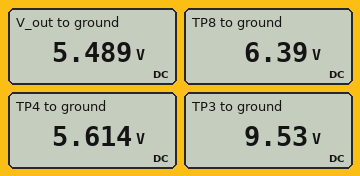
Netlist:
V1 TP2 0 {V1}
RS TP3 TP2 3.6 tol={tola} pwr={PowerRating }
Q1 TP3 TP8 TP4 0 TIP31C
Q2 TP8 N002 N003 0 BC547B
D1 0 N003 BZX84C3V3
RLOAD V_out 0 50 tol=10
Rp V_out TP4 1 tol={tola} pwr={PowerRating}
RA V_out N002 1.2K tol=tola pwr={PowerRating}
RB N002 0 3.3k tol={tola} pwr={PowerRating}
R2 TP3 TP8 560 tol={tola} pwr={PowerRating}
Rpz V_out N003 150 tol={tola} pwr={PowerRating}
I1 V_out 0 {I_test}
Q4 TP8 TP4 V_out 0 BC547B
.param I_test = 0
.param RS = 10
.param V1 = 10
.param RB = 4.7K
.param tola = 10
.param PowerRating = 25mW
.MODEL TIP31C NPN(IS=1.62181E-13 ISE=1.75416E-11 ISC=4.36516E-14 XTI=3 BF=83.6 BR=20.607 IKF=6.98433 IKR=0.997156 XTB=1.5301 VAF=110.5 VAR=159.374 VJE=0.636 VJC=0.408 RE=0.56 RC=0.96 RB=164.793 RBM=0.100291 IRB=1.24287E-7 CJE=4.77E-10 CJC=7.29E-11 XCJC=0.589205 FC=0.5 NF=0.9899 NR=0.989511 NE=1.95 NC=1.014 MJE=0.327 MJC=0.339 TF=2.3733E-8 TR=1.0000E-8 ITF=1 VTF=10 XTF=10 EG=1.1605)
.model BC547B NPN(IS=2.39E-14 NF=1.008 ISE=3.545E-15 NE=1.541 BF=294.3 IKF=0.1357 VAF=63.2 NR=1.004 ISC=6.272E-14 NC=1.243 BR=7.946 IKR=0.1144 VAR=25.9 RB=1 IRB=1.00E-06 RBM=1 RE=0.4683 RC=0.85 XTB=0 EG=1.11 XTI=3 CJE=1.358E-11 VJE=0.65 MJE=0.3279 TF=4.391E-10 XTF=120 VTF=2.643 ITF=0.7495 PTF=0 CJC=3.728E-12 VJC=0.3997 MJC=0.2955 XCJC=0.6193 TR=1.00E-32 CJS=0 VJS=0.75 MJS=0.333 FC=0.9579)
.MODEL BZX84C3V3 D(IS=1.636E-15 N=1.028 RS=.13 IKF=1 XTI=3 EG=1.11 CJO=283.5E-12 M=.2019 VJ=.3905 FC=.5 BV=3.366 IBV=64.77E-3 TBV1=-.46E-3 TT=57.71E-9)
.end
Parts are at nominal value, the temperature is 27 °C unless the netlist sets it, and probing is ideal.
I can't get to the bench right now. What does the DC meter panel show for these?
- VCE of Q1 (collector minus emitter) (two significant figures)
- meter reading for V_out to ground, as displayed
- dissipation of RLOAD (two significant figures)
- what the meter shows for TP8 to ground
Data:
3.9 V
5.489 V
600 mW
6.39 V
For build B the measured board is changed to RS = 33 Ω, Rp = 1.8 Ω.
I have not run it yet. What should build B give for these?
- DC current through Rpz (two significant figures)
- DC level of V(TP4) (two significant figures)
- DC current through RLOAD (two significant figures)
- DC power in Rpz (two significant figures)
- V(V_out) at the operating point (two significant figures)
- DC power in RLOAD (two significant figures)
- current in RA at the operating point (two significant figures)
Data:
9.9 mA
5.0 V
96 mA
15 mW
4.8 V
460 mW
1.1 mA
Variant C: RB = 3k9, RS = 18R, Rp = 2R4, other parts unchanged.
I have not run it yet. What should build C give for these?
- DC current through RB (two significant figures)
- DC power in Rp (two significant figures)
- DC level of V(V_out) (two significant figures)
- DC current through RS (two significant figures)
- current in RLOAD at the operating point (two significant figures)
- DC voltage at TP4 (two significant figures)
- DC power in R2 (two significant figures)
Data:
1.0 mA
33 mW
5.2 V
120 mA
100 mA
5.5 V
4.6 mW
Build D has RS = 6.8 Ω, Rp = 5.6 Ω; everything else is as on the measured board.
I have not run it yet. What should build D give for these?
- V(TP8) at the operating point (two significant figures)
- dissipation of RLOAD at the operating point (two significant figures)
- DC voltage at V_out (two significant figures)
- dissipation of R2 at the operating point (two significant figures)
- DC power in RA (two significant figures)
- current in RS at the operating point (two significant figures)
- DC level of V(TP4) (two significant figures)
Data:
6.8 V
570 mW
5.3 V
10 mW
1.7 mW
120 mA
6.0 V
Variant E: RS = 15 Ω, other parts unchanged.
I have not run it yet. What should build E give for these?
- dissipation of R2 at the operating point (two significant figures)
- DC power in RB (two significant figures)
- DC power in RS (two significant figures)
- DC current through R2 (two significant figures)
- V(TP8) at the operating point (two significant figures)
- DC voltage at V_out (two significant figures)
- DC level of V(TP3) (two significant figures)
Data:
5.7 mW
4.8 mW
240 mW
3.2 mA
6.3 V
5.4 V
8.1 V
